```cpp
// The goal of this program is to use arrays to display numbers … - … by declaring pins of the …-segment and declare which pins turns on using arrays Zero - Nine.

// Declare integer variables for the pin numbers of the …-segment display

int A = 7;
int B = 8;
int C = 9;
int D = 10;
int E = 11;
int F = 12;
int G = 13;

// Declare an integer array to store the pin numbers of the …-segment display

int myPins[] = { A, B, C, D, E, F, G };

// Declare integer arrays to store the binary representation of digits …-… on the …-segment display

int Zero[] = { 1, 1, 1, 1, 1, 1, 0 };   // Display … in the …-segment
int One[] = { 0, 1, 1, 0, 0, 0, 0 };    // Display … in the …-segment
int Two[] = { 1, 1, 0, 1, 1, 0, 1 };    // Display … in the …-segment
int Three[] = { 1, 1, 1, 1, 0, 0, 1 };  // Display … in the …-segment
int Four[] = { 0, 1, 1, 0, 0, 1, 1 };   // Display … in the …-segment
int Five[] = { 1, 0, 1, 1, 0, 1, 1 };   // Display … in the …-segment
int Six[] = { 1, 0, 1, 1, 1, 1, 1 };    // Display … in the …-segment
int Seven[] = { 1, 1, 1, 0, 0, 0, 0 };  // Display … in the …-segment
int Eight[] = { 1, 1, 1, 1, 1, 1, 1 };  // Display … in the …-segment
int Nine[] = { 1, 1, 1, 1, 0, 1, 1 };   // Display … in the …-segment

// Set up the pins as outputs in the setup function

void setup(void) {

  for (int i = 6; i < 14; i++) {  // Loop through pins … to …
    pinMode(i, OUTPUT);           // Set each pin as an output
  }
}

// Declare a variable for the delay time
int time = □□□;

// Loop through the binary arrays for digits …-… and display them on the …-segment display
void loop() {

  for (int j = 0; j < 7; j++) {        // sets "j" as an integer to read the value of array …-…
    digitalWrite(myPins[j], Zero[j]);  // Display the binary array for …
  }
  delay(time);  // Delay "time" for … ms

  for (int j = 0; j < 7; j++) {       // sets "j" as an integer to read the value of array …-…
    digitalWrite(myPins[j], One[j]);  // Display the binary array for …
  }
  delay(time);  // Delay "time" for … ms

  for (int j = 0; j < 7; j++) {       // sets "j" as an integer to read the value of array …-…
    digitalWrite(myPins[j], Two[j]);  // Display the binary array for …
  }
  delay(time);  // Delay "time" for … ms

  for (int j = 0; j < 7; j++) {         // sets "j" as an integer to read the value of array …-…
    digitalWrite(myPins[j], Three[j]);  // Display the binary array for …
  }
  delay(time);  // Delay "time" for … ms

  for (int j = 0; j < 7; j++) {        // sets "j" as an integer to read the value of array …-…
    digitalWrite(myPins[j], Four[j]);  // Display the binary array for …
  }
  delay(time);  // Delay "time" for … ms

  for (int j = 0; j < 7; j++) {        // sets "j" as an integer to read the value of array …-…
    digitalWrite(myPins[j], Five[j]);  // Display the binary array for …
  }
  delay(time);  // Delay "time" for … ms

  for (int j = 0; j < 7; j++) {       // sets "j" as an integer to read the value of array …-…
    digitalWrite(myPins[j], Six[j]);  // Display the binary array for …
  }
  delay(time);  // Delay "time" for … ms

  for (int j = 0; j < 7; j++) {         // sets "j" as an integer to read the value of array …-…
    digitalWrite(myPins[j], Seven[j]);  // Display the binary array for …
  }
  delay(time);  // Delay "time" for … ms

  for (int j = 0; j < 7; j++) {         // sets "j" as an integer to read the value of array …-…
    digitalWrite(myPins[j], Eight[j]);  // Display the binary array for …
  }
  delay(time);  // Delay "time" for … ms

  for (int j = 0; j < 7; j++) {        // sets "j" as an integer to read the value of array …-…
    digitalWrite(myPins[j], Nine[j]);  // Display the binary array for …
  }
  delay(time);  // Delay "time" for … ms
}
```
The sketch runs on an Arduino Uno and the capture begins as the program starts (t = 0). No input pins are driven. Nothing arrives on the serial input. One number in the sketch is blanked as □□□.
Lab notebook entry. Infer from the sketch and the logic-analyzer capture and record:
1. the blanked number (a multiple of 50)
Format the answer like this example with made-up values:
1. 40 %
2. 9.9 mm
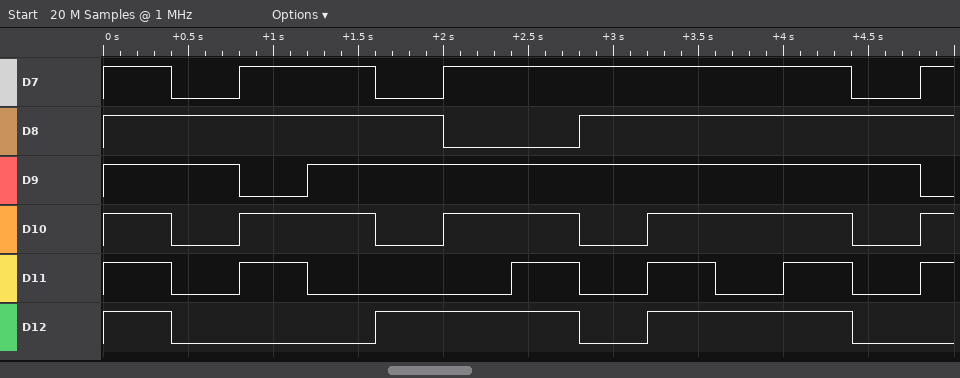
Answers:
1. 400
